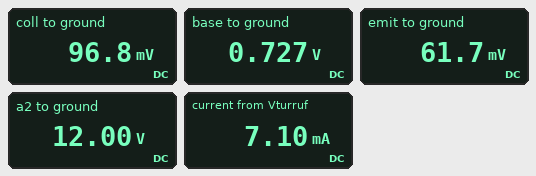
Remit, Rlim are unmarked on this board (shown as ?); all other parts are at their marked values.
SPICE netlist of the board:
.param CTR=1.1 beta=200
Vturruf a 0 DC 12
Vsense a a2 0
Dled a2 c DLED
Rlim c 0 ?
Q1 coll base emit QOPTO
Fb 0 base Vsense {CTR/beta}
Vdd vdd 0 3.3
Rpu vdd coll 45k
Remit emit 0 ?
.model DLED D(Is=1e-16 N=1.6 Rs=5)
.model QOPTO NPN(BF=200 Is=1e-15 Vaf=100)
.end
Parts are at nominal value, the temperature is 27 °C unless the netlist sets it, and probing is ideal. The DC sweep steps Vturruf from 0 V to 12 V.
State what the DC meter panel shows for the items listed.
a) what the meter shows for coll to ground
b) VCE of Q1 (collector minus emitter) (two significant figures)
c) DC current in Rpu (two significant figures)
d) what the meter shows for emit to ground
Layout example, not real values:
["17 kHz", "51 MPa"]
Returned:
["96.8 mV", "35 mV", "71 µA", "61.7 mV"]
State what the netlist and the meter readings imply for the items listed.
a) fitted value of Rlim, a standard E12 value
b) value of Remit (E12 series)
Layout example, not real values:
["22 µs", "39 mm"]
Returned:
["1.5 kΩ", "560 Ω"]
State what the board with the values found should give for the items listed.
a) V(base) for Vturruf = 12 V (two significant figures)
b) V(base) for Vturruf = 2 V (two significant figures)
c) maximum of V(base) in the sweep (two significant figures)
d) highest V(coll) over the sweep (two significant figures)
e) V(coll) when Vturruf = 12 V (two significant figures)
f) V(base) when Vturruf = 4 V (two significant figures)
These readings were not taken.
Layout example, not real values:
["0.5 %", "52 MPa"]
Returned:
["730 mV", "690 mV", "730 mV", "3.3 V", "97 mV", "700 mV"]
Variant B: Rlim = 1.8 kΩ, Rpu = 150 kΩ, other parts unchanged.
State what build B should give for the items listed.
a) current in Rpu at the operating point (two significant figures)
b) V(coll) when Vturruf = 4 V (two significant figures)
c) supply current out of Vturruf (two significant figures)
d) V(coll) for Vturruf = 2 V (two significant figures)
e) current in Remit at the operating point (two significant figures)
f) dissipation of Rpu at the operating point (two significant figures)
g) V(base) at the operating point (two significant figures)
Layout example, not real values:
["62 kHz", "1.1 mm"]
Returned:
["22 µA", "57 mV", "5.9 mA", "76 mV", "54 µA", "70 µW", "680 mV"]
